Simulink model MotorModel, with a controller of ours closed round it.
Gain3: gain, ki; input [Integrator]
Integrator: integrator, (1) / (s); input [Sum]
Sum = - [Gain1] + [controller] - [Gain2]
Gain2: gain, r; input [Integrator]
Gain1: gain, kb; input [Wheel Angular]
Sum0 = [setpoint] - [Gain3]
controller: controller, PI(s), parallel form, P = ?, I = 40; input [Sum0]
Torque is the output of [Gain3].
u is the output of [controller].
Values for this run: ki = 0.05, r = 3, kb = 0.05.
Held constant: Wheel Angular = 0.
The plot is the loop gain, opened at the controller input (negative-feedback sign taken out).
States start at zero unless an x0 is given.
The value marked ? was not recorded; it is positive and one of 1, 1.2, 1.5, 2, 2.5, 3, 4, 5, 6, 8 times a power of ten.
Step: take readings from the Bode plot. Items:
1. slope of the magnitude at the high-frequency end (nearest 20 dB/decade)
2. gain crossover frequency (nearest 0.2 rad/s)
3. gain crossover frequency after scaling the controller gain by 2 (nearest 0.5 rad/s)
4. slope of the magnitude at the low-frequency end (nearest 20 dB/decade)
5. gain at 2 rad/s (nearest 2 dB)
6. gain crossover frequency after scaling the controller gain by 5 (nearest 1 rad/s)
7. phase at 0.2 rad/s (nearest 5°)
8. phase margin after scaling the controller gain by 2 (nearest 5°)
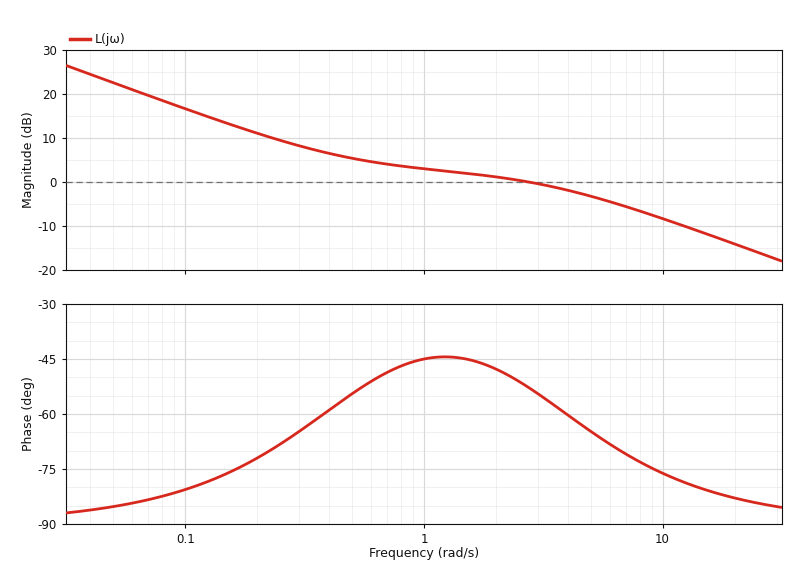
-20 dB/decade
2.8 rad/s
7.5 rad/s
-20 dB/decade
2 dB
20 rad/s
-70°
110°
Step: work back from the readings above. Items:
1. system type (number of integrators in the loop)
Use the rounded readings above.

1
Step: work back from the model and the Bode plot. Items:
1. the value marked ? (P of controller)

80
